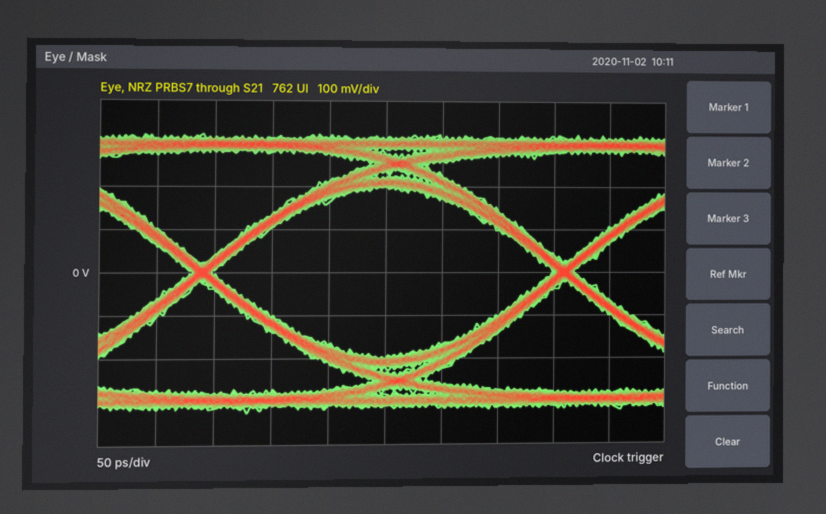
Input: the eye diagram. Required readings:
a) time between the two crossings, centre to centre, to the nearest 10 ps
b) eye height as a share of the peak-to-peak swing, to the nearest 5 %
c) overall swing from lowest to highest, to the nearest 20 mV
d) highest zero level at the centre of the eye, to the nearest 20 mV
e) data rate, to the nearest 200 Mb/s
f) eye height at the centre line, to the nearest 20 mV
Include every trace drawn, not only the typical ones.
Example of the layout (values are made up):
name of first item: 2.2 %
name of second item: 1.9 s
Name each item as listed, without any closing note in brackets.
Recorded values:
time between the two crossings, centre to centre, to the nearest 10 ps: 320 ps
eye height as a share of the peak-to-peak swing, to the nearest 5 %: 60 %
overall swing from lowest to highest, to the nearest 20 mV: 640 mV
highest zero level at the centre of the eye, to the nearest 20 mV: -200 mV
data rate, to the nearest 200 Mb/s: 3.2 Gb/s
eye height at the centre line, to the nearest 20 mV: 400 mV
